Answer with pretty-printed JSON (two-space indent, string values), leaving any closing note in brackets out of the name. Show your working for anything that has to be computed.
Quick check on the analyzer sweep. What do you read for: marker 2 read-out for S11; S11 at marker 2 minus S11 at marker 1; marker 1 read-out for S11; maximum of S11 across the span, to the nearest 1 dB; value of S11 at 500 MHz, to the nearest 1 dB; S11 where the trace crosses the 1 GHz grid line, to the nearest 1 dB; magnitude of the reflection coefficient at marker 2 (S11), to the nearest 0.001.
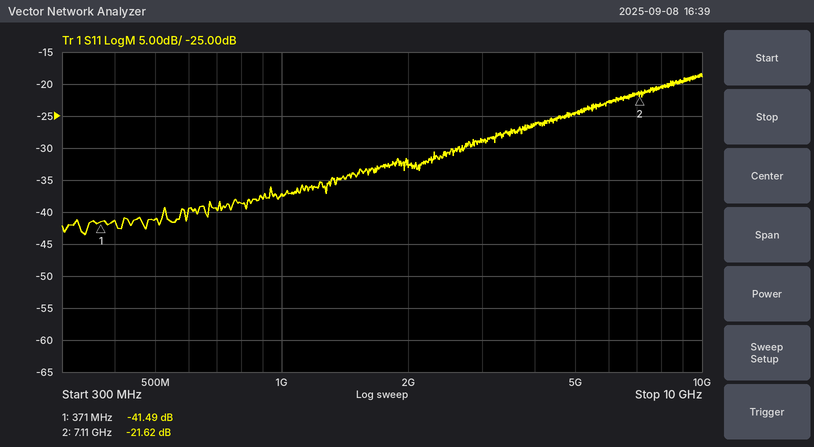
{
  "marker 2 read-out for S11": "-21.62 dB",
  "S11 at marker 2 minus S11 at marker 1": "-21.62 − (-41.49) = 19.87 dB",
  "marker 1 read-out for S11": "-41.49 dB",
  "maximum of S11 across the span, to the nearest 1 dB": "-18 dB",
  "value of S11 at 500 MHz, to the nearest 1 dB": "-41 dB",
  "S11 where the trace crosses the 1 GHz grid line, to the nearest 1 dB": "-37 dB",
  "magnitude of the reflection coefficient at marker 2 (S11), to the nearest 0.001": "10^(-21.62/20) ≈ 0.083"
}
